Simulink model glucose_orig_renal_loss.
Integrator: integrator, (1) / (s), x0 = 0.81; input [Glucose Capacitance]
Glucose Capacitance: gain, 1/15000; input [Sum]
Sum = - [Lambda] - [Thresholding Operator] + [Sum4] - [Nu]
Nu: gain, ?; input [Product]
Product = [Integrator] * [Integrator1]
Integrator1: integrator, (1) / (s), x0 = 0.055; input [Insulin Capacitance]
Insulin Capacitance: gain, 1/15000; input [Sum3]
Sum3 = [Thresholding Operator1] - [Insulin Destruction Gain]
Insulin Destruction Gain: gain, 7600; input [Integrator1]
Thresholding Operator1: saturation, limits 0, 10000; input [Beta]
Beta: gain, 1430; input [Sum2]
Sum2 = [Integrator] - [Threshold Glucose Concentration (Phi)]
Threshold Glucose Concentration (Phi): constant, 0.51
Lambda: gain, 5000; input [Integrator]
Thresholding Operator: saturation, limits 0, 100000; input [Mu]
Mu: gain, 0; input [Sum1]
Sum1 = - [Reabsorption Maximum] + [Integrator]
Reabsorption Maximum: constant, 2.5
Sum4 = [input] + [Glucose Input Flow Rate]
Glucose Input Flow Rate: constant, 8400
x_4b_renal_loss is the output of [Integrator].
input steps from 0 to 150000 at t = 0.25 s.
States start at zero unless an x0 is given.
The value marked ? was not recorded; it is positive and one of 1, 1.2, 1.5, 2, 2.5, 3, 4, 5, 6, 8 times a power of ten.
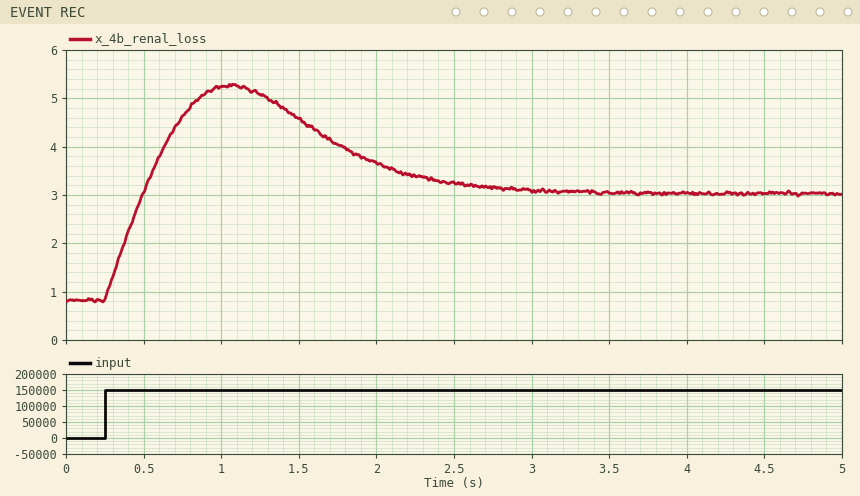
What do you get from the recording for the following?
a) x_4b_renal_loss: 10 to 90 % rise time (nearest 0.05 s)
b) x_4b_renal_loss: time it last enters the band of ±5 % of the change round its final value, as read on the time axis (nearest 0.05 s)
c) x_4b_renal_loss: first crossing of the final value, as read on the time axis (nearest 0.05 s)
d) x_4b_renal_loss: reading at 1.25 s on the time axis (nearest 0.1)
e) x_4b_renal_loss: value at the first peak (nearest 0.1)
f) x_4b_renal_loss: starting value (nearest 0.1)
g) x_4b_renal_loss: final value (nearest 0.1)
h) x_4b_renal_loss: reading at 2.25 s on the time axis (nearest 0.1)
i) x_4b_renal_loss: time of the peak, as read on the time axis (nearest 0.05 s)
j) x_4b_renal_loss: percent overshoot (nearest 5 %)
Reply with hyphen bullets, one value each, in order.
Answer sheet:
- 0.20 s
- 2.80 s
- 0.50 s
- 5.1
- 5.3
- 0.8
- 3.0
- 3.4
- 1.05 s
- 100 %
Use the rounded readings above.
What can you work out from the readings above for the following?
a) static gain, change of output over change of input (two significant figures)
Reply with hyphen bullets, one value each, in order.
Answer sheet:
- 0.000015
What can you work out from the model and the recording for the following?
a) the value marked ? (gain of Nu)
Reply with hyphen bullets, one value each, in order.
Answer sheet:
- 100000
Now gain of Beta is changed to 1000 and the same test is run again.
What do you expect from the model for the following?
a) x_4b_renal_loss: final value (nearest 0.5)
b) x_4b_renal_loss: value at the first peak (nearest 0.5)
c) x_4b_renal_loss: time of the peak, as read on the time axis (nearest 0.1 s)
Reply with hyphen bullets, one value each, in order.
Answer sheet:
- 3.5
- 6.0
- 1.2 s
